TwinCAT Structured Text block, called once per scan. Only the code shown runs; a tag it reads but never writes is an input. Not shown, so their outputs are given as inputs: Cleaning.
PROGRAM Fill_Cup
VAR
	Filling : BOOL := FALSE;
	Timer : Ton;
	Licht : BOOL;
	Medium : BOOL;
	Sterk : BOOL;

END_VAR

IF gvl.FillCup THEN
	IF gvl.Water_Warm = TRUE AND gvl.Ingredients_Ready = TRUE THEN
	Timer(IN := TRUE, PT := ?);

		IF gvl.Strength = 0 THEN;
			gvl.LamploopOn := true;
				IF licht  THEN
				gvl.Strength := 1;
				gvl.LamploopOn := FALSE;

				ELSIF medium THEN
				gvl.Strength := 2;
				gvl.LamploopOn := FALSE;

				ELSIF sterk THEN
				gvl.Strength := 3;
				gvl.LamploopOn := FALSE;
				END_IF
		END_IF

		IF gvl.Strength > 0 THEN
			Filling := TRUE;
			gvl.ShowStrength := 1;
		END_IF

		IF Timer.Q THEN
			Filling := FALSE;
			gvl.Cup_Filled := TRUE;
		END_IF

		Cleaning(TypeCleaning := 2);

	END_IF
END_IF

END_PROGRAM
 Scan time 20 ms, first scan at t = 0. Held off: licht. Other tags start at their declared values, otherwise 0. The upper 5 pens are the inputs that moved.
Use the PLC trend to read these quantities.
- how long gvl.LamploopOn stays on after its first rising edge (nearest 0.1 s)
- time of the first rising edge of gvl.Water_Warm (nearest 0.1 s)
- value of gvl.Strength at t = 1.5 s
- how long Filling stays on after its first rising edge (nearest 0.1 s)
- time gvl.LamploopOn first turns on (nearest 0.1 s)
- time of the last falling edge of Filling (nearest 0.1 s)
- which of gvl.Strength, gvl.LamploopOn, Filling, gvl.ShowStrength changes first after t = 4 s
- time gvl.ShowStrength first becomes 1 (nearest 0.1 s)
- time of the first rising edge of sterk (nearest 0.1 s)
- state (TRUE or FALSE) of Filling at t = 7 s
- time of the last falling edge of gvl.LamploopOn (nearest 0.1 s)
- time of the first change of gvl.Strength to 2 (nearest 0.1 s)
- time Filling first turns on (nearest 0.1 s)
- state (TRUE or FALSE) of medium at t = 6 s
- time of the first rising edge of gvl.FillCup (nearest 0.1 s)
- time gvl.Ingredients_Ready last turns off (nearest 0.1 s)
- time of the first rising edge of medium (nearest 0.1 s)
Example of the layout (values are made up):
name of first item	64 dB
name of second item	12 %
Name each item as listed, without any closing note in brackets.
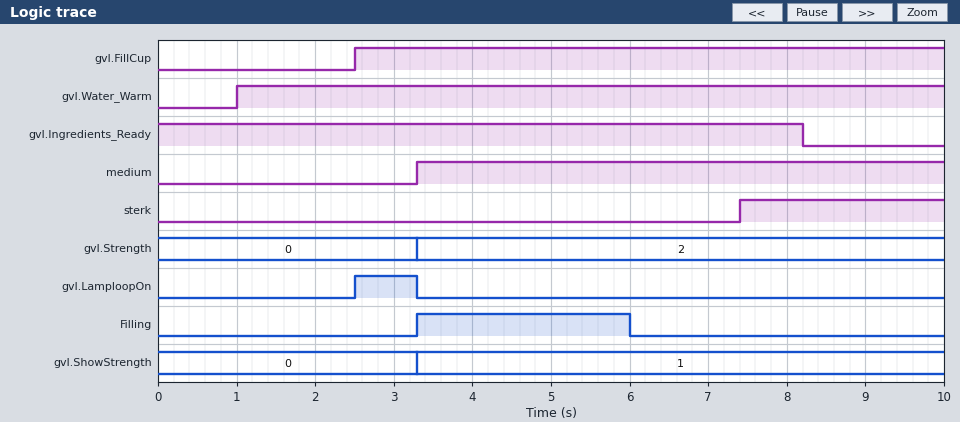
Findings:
how long gvl.LamploopOn stays on after its first rising edge	0.8 s
time of the first rising edge of gvl.Water_Warm	1.0 s
value of gvl.Strength at t = 1.5 s	0
how long Filling stays on after its first rising edge	2.7 s
time gvl.LamploopOn first turns on	2.5 s
time of the last falling edge of Filling	6.0 s
which of gvl.Strength, gvl.LamploopOn, Filling, gvl.ShowStrength changes first after t = 4 s	Filling
time gvl.ShowStrength first becomes 1	3.3 s
time of the first rising edge of sterk	7.4 s
state (TRUE or FALSE) of Filling at t = 7 s	FALSE
time of the last falling edge of gvl.LamploopOn	3.3 s
time of the first change of gvl.Strength to 2	3.3 s
time Filling first turns on	3.3 s
state (TRUE or FALSE) of medium at t = 6 s	TRUE
time of the first rising edge of gvl.FillCup	2.5 s
time gvl.Ingredients_Ready last turns off	8.2 s
time of the first rising edge of medium	3.3 s
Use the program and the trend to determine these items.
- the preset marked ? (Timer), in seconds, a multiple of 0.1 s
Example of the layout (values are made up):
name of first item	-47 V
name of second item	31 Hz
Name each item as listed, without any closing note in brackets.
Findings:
the preset marked ? (Timer), in seconds, a multiple of 0.1 s	3.5 s
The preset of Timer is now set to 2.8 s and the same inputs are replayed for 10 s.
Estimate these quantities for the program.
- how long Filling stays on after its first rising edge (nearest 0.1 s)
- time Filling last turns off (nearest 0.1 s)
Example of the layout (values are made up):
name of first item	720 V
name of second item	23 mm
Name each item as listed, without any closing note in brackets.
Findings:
how long Filling stays on after its first rising edge	2.0 s
time Filling last turns off	5.3 s
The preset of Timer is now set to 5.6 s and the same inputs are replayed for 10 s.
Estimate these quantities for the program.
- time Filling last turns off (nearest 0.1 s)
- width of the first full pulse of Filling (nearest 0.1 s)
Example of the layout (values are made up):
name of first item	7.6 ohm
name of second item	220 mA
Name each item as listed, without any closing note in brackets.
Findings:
time Filling last turns off	8.1 s
width of the first full pulse of Filling	4.8 s
